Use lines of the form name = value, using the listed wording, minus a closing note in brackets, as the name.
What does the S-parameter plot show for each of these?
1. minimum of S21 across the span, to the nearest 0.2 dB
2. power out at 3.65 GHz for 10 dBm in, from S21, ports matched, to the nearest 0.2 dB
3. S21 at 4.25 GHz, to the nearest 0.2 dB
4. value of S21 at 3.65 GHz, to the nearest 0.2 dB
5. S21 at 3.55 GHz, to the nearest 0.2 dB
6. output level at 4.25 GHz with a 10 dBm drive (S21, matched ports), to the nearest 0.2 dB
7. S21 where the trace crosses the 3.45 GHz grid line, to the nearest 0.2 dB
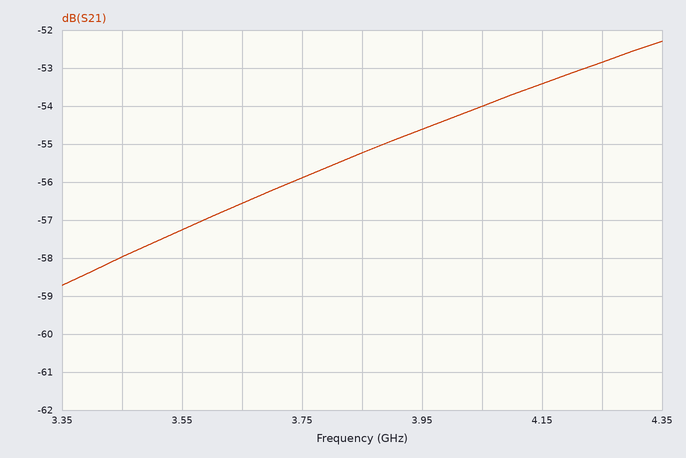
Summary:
minimum of S21 across the span, to the nearest 0.2 dB = -58.8 dB
power out at 3.65 GHz for 10 dBm in, from S21, ports matched, to the nearest 0.2 dB = -46.6 dBm
S21 at 4.25 GHz, to the nearest 0.2 dB = -52.8 dB
value of S21 at 3.65 GHz, to the nearest 0.2 dB = -56.6 dB
S21 at 3.55 GHz, to the nearest 0.2 dB = -57.2 dB
output level at 4.25 GHz with a 10 dBm drive (S21, matched ports), to the nearest 0.2 dB = -42.8 dBm
S21 where the trace crosses the 3.45 GHz grid line, to the nearest 0.2 dB = -58.0 dB
